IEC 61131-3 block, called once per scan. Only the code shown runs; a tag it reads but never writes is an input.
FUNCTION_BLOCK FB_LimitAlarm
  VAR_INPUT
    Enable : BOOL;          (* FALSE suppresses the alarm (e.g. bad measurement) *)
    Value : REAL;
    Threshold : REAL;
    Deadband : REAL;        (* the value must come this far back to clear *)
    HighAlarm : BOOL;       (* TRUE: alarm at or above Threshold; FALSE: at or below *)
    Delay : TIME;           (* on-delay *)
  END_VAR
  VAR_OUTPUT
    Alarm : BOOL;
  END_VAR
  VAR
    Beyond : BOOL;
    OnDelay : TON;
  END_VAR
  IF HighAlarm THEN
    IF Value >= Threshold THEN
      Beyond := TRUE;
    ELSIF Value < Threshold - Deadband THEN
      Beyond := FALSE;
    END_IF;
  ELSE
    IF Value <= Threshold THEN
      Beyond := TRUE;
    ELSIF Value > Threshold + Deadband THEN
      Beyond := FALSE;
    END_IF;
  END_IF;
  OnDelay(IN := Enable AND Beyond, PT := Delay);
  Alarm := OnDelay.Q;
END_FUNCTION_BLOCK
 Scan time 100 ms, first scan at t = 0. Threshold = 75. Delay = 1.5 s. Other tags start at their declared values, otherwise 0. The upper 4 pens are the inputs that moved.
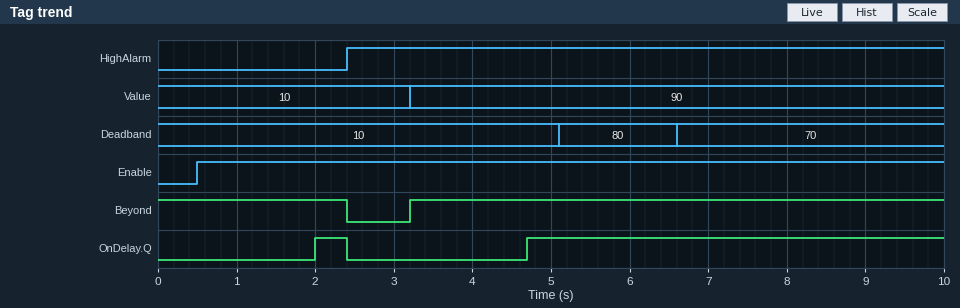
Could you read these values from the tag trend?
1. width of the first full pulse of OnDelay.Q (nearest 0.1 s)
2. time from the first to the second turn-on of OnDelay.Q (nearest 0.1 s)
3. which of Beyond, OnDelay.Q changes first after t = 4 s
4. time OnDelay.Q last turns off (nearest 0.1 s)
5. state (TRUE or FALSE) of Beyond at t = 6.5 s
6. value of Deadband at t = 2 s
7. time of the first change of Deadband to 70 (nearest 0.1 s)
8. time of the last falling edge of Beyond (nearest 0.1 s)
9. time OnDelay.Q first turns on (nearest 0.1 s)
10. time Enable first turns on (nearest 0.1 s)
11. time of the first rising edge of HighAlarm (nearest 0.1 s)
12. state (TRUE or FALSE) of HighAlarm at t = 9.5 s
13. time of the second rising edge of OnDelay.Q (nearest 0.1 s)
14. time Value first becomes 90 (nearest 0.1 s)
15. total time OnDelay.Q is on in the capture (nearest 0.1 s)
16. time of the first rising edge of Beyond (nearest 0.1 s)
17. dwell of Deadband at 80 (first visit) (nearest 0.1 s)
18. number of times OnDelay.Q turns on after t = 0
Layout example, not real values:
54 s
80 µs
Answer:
0.4 s
2.7 s
OnDelay.Q
2.4 s
TRUE
10
6.6 s
2.4 s
2.0 s
0.5 s
2.4 s
TRUE
4.7 s
3.2 s
5.7 s
3.2 s
1.5 s
2
